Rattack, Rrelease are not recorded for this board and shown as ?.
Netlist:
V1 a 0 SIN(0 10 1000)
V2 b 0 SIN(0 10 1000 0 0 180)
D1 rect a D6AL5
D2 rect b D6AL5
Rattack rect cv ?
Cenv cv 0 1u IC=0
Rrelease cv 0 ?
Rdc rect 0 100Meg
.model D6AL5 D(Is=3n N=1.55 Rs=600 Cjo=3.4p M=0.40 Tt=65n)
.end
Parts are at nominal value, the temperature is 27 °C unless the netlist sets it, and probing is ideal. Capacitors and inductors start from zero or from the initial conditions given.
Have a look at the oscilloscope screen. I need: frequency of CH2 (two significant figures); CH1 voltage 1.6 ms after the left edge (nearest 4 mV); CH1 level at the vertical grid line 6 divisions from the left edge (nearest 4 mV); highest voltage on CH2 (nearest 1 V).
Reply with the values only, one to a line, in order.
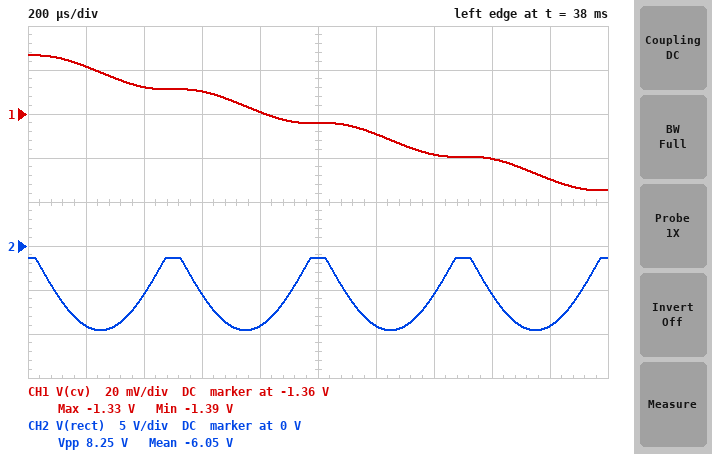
2.0 kHz
-1.380 V
-1.368 V
-1 V
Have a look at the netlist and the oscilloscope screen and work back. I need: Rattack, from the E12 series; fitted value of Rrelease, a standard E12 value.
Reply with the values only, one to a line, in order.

150 kΩ
1.8 MΩ
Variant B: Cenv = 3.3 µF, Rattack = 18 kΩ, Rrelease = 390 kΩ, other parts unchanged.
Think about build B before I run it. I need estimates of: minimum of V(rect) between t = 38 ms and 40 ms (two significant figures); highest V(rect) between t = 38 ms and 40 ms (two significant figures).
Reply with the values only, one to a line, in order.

-9.3 V
-2.8 V
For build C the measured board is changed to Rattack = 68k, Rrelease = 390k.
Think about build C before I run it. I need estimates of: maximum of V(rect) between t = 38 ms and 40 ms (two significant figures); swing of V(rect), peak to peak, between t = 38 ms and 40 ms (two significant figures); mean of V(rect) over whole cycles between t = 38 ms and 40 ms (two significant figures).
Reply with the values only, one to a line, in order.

-2.5 V
7.0 V
-6.2 V
